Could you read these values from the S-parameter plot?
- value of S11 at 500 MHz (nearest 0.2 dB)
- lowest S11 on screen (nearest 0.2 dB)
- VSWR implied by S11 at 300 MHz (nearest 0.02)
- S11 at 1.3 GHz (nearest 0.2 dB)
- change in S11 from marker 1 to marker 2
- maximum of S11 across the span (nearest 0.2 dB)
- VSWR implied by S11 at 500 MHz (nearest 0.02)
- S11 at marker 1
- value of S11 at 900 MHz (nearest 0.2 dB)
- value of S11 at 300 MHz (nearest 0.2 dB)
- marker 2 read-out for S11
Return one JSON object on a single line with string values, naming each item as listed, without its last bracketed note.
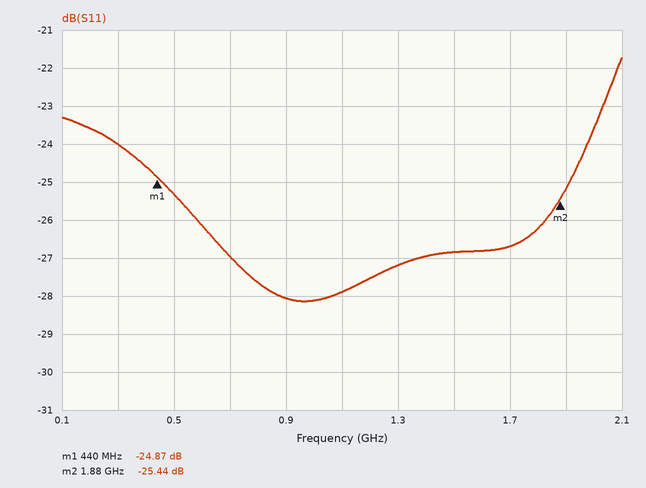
{"value of S11 at 500 MHz": "-25.4 dB", "lowest S11 on screen": "-28.2 dB", "VSWR implied by S11 at 300 MHz": "1.14", "S11 at 1.3 GHz": "-27.2 dB", "change in S11 from marker 1 to marker 2": "-0.57 dB", "maximum of S11 across the span": "-21.8 dB", "VSWR implied by S11 at 500 MHz": "1.12", "S11 at marker 1": "-24.87 dB", "value of S11 at 900 MHz": "-28.0 dB", "value of S11 at 300 MHz": "-24.0 dB", "marker 2 read-out for S11": "-25.44 dB"}
